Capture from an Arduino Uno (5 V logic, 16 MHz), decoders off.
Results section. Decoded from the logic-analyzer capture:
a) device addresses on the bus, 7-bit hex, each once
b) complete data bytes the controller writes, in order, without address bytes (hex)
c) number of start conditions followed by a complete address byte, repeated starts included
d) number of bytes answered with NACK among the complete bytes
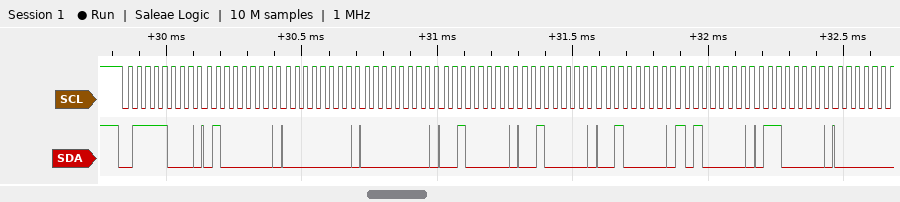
0x3C
40 00 00 20 20 20 A0 60
1
0
